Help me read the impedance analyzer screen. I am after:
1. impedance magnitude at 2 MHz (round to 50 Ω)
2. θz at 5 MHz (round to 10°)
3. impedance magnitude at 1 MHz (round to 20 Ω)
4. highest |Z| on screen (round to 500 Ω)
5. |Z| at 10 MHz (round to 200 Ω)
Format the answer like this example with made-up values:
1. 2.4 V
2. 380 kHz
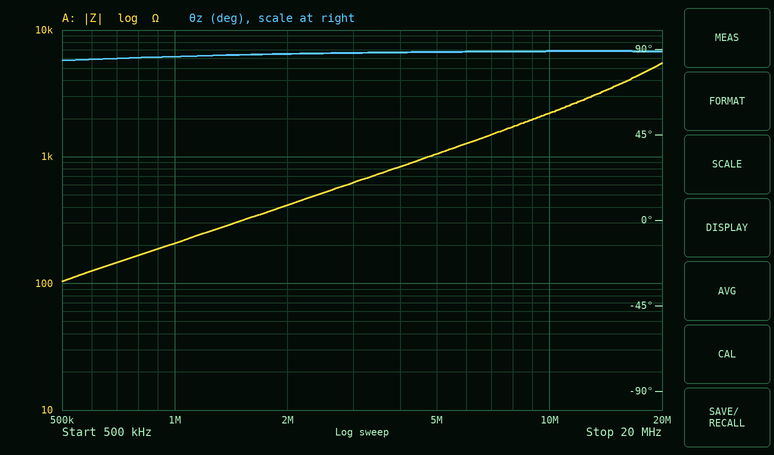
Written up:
1. 400 Ω
2. 90°
3. 200 Ω
4. 5.5 kΩ
5. 2.2 kΩ
